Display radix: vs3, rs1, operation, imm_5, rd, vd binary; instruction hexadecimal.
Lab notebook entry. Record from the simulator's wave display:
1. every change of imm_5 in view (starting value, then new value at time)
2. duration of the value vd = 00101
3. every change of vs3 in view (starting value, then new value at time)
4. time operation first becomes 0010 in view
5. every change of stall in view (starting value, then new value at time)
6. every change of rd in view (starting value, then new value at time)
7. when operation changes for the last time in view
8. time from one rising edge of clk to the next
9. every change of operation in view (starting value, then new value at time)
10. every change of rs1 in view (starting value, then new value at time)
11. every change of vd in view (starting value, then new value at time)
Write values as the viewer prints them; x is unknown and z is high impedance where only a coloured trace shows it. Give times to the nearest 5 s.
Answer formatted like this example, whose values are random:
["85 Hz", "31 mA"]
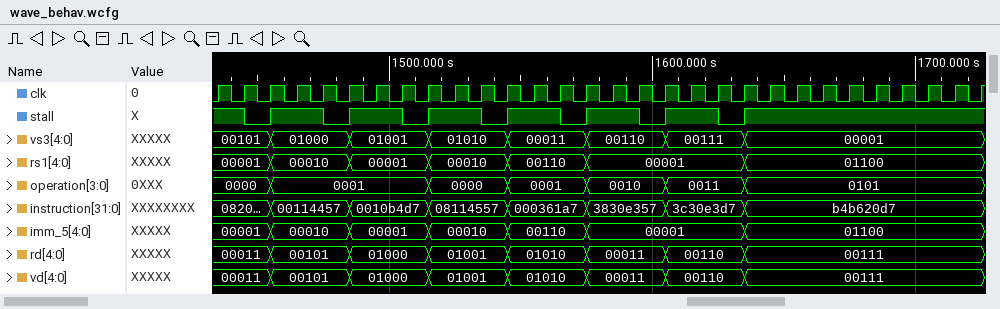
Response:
["00001, 00010 at 1455 s, 00001 at 1485 s, 00010 at 1515 s, 00110 at 1545 s, 00001 at 1575 s, 01100 at 1635 s", "30 s", "00101, 01000 at 1455 s, 01001 at 1485 s, 01010 at 1515 s, 00011 at 1545 s, 00110 at 1575 s, 00111 at 1605 s, 00001 at 1635 s", "1575 s", "1, 0 at 1445 s, 1 at 1455 s, 0 at 1475 s, 1 at 1485 s, 0 at 1505 s, 1 at 1515 s, 0 at 1535 s, 1 at 1545 s, 0 at 1565 s, 1 at 1575 s, 0 at 1595 s, 1 at 1605 s, 0 at 1625 s, 1 at 1635 s", "00011, 00101 at 1455 s, 01000 at 1485 s, 01001 at 1515 s, 01010 at 1545 s, 00011 at 1575 s, 00110 at 1605 s, 00111 at 1635 s", "1635 s", "10 s", "0000, 0001 at 1455 s, 0000 at 1515 s, 0001 at 1545 s, 0010 at 1575 s, 0011 at 1605 s, 0101 at 1635 s", "00001, 00010 at 1455 s, 00001 at 1485 s, 00010 at 1515 s, 00110 at 1545 s, 00001 at 1575 s, 01100 at 1635 s", "00011, 00101 at 1455 s, 01000 at 1485 s, 01001 at 1515 s, 01010 at 1545 s, 00011 at 1575 s, 00110 at 1605 s, 00111 at 1635 s"]
